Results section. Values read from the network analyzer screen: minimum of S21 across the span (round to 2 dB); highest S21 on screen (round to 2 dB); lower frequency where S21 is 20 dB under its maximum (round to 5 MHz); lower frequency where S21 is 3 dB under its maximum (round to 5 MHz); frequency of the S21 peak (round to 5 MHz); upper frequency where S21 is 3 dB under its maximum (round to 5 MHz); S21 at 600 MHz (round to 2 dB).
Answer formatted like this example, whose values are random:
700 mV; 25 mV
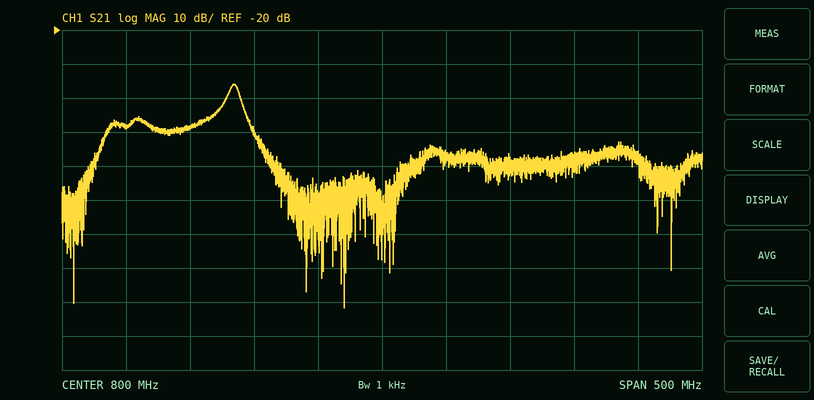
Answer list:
-102 dB; -36 dB; 580 MHz; 680 MHz; 685 MHz; 690 MHz; -48 dB
